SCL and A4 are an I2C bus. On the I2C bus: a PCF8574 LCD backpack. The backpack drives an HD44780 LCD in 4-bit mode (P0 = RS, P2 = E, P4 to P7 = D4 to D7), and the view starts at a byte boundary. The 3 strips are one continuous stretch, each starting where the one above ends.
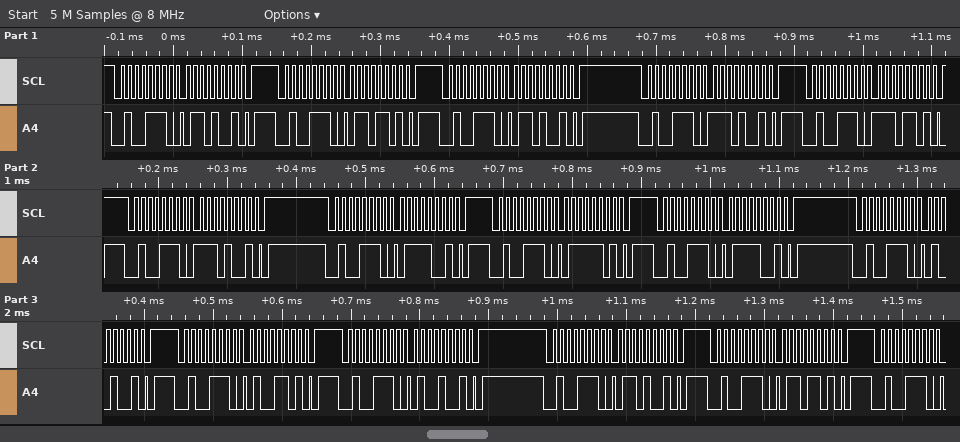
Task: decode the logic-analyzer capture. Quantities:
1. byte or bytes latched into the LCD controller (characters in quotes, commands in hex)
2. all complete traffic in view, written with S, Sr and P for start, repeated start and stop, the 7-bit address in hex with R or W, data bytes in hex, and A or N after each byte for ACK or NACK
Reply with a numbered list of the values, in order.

1. 'n' 't'
2. S 27W A 69 A P S 27W A 6D A P S 27W A 69 A P S 27W A E9 A P S 27W A ED A P S 27W A E9 A P S 27W A 79 A P S 27W A 7D A P S 27W A 79 A P S 27W A 49 A P S 27W A 4D A P S 27W A 49 A P S 27W A 69 A P S 27W A 6D A P S 27W A
